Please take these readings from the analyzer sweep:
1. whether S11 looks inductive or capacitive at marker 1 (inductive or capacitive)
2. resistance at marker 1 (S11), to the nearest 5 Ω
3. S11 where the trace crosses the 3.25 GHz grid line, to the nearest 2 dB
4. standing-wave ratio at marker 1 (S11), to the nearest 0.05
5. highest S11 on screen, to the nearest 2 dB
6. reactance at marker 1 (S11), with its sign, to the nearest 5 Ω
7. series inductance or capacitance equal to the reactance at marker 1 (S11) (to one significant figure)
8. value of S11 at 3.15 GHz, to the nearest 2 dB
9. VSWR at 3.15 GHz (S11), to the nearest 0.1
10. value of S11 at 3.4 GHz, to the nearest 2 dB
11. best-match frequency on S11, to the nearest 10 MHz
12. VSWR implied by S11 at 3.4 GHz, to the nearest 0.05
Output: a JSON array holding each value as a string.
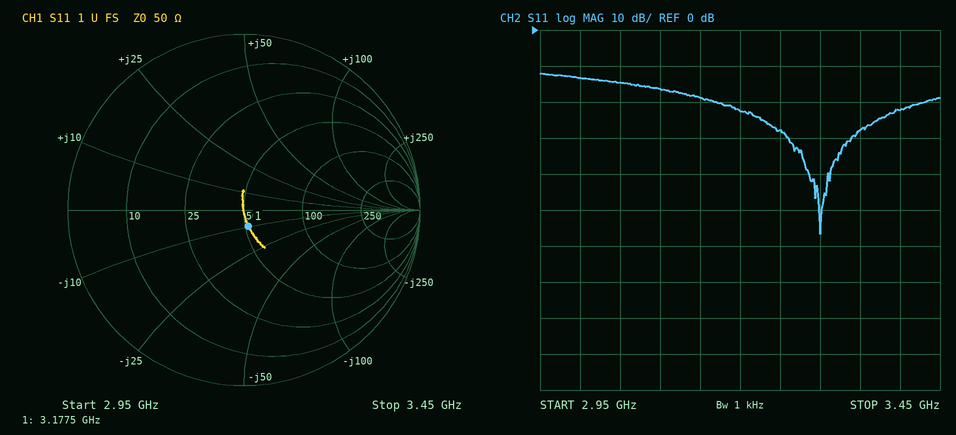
["capacitive", "50 Ω", "-28 dB", "1.20", "-12 dB", "-10 Ω", "5 pF", "-18 dB", "1.3", "-22 dB", "3.30 GHz", "1.15"]
